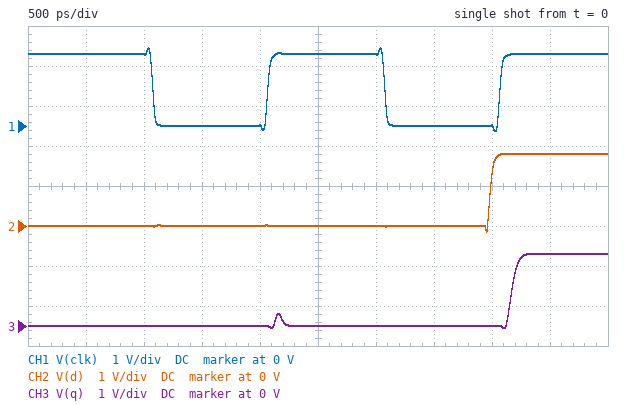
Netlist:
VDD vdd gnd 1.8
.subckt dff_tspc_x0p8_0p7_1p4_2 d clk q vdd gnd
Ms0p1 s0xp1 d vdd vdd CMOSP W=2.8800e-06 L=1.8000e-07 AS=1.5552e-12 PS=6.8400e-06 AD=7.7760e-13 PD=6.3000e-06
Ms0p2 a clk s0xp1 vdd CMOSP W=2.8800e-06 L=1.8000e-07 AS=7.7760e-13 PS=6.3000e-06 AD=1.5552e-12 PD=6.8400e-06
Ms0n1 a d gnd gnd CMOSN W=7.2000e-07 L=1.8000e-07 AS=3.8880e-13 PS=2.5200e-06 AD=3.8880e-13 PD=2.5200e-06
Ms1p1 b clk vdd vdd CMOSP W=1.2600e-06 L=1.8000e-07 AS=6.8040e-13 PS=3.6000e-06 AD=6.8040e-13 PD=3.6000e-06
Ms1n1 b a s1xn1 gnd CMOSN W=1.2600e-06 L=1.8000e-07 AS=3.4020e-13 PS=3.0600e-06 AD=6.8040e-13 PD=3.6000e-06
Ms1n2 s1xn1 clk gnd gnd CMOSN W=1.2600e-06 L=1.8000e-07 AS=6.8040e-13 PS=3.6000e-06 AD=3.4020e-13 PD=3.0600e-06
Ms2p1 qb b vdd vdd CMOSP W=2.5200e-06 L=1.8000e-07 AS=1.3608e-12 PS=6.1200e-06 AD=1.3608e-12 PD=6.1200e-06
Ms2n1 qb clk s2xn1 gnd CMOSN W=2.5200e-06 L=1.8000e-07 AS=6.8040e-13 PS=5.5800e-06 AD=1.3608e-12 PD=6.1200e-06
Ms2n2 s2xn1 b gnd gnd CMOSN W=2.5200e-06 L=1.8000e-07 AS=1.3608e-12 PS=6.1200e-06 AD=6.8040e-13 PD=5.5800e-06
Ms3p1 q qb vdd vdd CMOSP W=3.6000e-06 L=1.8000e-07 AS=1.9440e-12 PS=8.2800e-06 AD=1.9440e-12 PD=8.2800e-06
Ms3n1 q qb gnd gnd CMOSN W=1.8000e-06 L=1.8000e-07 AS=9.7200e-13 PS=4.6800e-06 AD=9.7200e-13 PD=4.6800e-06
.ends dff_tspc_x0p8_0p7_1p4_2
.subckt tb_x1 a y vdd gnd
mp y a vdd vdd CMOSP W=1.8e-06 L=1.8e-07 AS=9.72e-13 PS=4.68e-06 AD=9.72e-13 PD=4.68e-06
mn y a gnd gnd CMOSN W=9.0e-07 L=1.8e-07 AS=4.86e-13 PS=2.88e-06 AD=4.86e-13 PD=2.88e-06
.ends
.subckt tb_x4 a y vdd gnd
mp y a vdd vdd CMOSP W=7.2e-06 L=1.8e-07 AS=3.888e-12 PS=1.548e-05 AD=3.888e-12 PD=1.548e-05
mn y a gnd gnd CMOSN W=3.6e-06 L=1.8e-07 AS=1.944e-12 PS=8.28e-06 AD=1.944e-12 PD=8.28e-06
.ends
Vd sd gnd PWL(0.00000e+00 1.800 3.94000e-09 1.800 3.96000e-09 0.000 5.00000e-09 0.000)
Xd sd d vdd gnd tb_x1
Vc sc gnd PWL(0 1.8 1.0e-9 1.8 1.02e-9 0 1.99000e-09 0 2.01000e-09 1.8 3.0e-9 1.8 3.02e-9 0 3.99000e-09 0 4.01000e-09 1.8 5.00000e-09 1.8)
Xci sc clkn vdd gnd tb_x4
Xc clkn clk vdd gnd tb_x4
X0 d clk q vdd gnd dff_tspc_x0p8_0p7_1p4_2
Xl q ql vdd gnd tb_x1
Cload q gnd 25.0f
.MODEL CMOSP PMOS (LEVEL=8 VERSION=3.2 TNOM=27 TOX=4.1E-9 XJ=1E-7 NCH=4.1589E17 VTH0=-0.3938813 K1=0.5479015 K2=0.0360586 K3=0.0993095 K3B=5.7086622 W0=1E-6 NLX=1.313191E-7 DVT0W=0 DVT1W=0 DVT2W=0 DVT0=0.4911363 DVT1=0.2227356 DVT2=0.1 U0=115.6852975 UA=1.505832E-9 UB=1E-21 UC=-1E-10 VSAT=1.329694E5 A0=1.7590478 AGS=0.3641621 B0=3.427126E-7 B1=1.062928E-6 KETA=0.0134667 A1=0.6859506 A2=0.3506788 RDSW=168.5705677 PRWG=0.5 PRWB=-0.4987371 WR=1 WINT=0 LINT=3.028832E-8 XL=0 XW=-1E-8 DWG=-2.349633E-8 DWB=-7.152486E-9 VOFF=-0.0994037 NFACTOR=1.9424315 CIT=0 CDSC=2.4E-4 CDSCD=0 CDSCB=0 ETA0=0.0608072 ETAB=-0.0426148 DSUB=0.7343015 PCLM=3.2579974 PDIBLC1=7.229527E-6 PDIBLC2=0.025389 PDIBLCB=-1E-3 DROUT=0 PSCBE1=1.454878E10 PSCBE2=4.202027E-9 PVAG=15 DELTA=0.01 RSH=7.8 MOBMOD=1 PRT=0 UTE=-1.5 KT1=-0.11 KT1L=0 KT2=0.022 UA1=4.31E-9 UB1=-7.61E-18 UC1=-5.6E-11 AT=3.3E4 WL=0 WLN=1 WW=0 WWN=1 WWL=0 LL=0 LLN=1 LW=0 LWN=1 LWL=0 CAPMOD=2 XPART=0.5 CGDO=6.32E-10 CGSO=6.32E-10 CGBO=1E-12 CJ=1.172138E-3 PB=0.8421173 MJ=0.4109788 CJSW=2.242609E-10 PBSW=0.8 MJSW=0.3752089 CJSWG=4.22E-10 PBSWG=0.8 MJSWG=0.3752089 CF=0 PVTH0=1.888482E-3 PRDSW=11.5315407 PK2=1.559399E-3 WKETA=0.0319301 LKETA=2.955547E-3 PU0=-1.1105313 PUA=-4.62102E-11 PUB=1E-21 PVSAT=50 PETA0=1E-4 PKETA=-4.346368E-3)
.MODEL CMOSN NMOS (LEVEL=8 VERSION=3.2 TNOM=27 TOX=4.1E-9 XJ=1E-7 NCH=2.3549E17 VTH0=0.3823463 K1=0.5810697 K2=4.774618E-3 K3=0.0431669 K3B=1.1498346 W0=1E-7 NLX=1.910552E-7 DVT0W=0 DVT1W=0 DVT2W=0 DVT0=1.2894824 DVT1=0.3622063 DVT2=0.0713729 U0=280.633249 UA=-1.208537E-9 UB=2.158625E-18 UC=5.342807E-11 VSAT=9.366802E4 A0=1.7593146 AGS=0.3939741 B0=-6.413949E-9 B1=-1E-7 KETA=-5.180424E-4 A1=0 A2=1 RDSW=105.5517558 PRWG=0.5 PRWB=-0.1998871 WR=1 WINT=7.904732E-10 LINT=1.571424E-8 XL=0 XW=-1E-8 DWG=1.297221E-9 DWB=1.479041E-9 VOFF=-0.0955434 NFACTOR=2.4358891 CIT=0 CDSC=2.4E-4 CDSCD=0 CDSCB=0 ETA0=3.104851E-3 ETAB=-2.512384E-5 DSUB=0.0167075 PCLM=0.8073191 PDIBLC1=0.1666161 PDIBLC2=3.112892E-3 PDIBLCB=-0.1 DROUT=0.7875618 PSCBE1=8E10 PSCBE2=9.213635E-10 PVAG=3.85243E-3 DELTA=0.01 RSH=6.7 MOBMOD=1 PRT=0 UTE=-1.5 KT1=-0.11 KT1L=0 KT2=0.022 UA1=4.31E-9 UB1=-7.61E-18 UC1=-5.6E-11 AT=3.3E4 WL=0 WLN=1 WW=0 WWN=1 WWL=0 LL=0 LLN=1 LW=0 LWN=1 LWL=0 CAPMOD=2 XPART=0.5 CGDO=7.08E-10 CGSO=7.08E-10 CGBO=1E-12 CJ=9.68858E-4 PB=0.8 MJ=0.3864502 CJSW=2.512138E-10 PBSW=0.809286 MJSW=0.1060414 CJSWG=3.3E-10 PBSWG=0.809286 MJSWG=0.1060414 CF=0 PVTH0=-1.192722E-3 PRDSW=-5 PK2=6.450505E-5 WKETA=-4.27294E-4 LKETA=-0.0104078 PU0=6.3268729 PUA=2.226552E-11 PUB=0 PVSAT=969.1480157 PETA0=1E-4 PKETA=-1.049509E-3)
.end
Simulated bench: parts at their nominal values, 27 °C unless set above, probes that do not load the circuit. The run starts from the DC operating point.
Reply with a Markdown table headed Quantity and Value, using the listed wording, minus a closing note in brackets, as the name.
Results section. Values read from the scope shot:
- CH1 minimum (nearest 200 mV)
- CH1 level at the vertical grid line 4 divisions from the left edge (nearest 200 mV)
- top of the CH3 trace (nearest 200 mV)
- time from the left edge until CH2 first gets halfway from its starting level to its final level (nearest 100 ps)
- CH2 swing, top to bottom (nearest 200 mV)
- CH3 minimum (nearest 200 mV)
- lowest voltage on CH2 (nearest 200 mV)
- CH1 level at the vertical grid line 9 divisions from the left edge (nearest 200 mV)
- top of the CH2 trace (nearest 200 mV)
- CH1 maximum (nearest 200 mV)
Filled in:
| Quantity | Value |
|---|---|
| CH1 minimum | -200 mV |
| CH1 level at the vertical grid line 4 divisions from the left edge | 0 V |
| top of the CH3 trace | 1.8 V |
| time from the left edge until CH2 first gets halfway from its starting level to its final level | 4.0 ns |
| CH2 swing, top to bottom | 2.0 V |
| CH3 minimum | 0 V |
| lowest voltage on CH2 | -200 mV |
| CH1 level at the vertical grid line 9 divisions from the left edge | 1.8 V |
| top of the CH2 trace | 1.8 V |
| CH1 maximum | 2.0 V |
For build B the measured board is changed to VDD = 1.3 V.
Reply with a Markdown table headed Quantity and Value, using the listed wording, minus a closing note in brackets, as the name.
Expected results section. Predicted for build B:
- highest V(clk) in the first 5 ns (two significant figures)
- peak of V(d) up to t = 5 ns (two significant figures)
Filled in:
| Quantity | Value |
|---|---|
| highest V(clk) in the first 5 ns | 1.4 V |
| peak of V(d) up to t = 5 ns | 1.3 V |
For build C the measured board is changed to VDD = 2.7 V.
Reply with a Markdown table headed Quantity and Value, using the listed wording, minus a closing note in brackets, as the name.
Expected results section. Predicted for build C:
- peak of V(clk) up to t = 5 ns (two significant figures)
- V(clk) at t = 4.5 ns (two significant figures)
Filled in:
| Quantity | Value |
|---|---|
| peak of V(clk) up to t = 5 ns | 2.9 V |
| V(clk) at t = 4.5 ns | 2.7 V |
